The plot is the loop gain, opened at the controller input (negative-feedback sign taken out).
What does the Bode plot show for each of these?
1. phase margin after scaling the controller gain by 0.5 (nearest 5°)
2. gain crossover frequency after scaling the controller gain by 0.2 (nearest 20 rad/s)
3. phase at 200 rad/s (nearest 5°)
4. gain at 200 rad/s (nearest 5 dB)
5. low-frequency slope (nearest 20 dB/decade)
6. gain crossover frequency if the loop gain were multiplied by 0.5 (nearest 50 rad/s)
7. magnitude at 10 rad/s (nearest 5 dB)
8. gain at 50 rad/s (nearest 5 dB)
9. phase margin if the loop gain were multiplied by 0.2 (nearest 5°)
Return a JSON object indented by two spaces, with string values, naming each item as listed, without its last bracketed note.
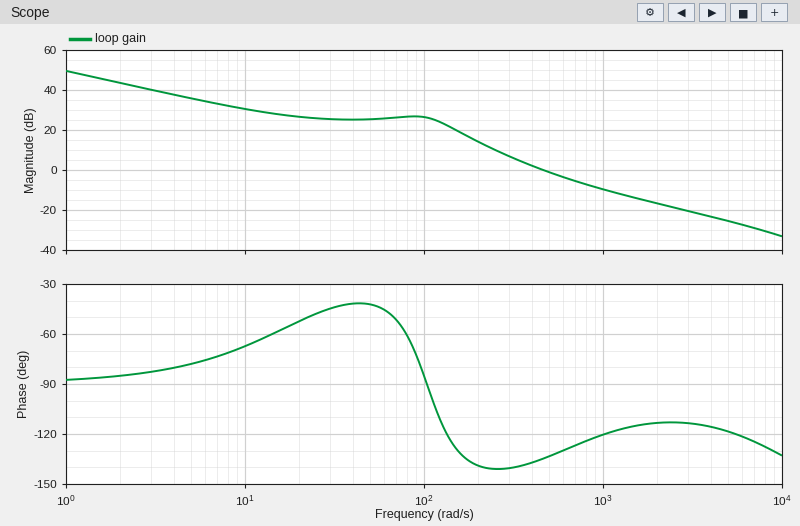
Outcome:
{
  "phase margin after scaling the controller gain by 0.5": "40°",
  "gain crossover frequency after scaling the controller gain by 0.2": "200 rad/s",
  "phase at 200 rad/s": "-140°",
  "gain at 200 rad/s": "15 dB",
  "low-frequency slope": "-20 dB/decade",
  "gain crossover frequency if the loop gain were multiplied by 0.5": "300 rad/s",
  "magnitude at 10 rad/s": "30 dB",
  "gain at 50 rad/s": "25 dB",
  "phase margin if the loop gain were multiplied by 0.2": "40°"
}
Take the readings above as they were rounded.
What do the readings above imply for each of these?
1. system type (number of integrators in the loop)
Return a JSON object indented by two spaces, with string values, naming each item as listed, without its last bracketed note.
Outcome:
{
  "system type": "1"
}
